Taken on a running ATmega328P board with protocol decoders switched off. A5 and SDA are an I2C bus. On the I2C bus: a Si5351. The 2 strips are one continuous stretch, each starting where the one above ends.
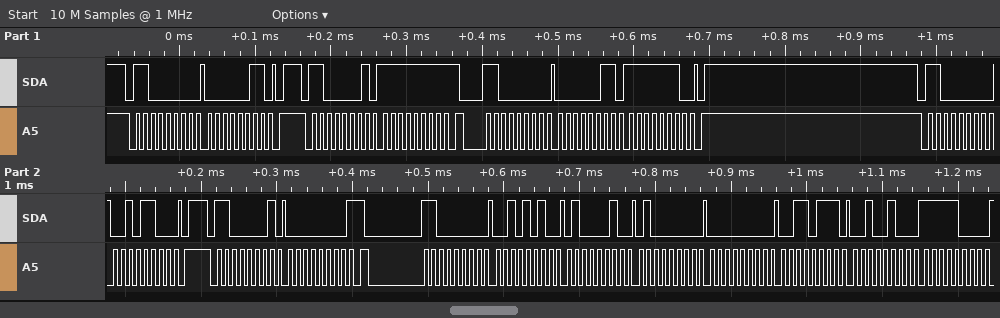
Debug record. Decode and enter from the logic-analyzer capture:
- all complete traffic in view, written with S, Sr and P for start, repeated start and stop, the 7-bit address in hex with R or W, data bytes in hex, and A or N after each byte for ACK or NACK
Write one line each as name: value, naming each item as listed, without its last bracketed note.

all complete traffic in view, written with S, Sr and P for start, repeated start and stop, the 7-bit address in hex with R or W, data bytes in hex, and A or N after each byte for ACK or NACK: S 60W A 03 A P S 60R A FF N Sr 60W A 03 A FE A P S 60W A 2C A P S 60R A 00 N Sr 60W A 2A A 42 A 40 A 00 A 37 A 24 A F8 A
